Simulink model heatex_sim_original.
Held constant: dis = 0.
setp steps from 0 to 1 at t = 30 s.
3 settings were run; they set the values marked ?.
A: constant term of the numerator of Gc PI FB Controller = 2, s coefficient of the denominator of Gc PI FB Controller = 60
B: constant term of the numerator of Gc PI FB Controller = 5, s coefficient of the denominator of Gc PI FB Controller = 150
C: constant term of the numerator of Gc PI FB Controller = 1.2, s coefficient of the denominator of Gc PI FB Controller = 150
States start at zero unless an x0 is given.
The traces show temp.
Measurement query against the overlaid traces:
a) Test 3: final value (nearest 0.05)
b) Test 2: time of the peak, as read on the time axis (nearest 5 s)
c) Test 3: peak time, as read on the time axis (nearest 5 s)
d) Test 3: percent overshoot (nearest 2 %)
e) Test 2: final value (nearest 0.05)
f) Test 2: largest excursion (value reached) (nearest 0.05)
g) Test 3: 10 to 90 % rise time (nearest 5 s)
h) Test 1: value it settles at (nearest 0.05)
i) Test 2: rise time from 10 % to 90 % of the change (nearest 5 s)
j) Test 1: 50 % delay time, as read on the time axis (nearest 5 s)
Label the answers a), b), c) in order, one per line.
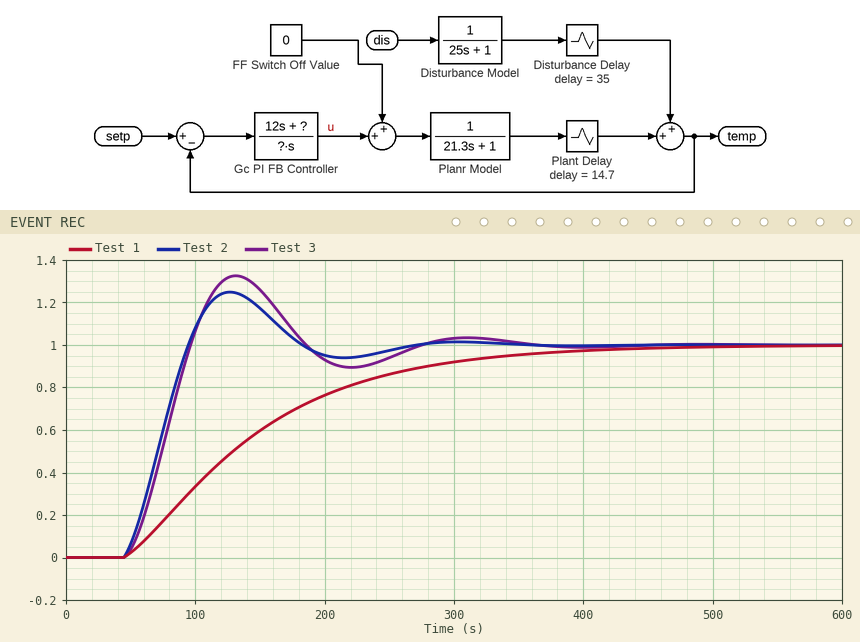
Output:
a) 1.00
b) 125 s
c) 130 s
d) 32 %
e) 1.00
f) 1.25
g) 35 s
h) 1.00
i) 35 s
j) 130 s
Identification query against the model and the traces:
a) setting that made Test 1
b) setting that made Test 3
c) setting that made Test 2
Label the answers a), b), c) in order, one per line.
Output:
a) C
b) B
c) A
